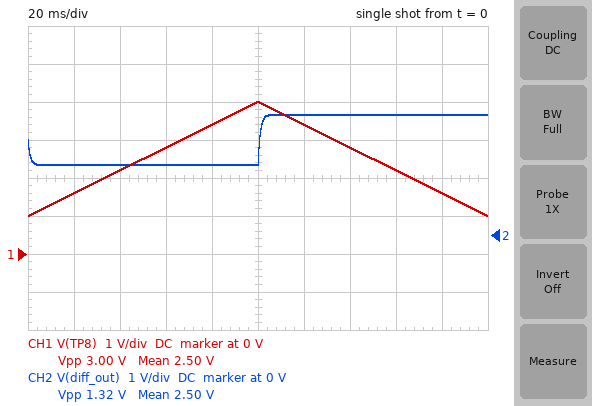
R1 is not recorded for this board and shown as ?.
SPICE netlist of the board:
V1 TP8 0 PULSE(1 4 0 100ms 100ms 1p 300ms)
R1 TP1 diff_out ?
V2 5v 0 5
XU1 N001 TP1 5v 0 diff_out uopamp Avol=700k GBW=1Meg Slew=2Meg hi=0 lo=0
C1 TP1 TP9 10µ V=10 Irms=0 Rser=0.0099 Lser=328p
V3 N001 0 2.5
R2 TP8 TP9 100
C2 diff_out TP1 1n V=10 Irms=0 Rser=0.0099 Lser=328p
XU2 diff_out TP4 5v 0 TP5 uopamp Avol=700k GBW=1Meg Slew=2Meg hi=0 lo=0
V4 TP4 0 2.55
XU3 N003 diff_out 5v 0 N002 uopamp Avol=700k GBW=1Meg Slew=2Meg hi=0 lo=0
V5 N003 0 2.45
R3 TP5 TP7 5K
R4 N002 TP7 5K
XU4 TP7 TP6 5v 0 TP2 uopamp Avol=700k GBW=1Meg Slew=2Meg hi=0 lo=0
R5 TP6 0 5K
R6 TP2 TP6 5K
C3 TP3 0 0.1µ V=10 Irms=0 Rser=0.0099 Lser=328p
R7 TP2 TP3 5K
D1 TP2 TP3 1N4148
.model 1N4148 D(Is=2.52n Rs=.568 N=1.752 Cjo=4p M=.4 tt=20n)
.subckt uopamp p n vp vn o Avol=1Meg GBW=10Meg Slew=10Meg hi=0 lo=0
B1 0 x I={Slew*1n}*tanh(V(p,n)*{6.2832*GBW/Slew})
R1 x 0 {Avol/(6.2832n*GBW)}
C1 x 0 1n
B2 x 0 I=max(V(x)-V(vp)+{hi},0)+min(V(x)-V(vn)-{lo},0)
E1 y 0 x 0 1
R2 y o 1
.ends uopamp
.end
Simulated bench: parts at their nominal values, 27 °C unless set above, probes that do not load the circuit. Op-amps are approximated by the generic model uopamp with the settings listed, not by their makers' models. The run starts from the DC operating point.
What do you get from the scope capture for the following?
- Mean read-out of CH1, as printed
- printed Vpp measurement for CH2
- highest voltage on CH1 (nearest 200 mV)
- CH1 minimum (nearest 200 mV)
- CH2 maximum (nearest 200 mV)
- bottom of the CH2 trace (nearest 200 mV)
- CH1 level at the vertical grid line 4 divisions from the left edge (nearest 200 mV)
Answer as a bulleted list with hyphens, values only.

- 2.50 V
- 1.32 V
- 4.0 V
- 1.0 V
- 3.2 V
- 1.8 V
- 3.4 V
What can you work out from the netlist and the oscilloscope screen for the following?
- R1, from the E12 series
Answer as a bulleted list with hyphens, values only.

- 2.2 kΩ
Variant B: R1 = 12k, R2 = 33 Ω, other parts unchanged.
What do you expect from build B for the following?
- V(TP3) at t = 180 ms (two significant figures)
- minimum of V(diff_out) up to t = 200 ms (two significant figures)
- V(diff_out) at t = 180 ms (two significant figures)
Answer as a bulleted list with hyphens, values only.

- 5.0 V
- -1.7 mV
- 5.0 V
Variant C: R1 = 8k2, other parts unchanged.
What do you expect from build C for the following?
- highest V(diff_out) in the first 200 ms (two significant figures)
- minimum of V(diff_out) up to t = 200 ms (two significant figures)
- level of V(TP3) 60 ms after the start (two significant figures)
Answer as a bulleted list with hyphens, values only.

- 5.0 V
- 40 mV
- 5.0 V
